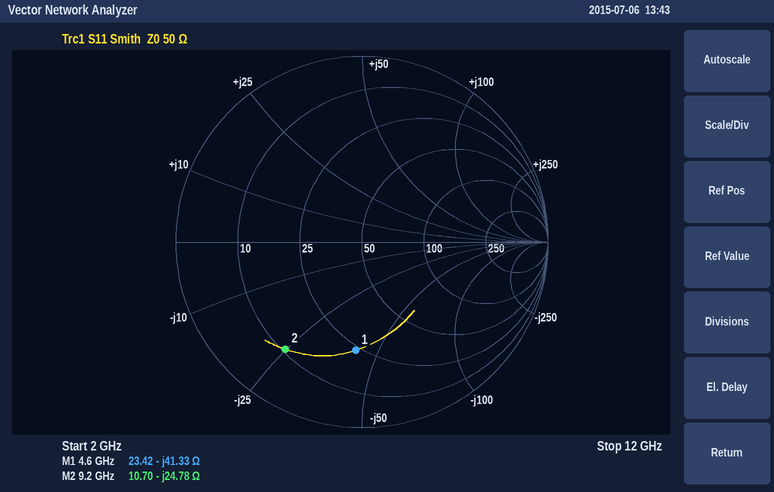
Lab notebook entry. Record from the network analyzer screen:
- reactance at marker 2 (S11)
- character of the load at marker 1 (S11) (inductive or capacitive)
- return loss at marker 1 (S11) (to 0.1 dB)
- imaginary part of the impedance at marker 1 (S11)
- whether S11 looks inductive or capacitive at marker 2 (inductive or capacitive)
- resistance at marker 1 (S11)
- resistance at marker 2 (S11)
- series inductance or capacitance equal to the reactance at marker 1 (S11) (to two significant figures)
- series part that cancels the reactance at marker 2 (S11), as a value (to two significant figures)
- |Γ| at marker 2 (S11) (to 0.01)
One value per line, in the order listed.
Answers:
-24.78 Ω
capacitive
4.7 dB
-41.33 Ω
capacitive
23.42 Ω
10.70 Ω
840 fF
430 pH
0.71
